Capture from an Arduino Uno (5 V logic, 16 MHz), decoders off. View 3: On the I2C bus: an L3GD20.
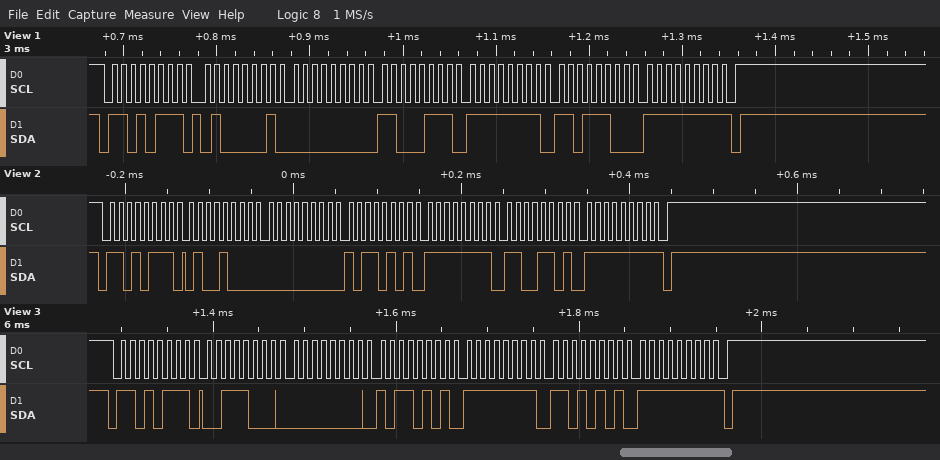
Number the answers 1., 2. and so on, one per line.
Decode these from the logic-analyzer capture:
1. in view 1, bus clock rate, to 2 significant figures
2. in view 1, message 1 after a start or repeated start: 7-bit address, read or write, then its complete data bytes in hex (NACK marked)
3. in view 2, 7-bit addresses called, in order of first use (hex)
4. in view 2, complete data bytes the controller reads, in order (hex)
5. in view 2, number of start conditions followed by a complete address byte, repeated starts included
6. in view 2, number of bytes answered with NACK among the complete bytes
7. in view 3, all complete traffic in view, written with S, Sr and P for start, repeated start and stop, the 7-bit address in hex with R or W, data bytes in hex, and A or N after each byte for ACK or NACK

1. 100 kHz
2. 0x6B read: 41 00 C7 FF DC FF NACK
3. 0x6B
4. 48 00 B5 FF CD FF
5. 1
6. 1
7. S 6BR A 38 A 00 A B5 A FF A D5 A FF N P
